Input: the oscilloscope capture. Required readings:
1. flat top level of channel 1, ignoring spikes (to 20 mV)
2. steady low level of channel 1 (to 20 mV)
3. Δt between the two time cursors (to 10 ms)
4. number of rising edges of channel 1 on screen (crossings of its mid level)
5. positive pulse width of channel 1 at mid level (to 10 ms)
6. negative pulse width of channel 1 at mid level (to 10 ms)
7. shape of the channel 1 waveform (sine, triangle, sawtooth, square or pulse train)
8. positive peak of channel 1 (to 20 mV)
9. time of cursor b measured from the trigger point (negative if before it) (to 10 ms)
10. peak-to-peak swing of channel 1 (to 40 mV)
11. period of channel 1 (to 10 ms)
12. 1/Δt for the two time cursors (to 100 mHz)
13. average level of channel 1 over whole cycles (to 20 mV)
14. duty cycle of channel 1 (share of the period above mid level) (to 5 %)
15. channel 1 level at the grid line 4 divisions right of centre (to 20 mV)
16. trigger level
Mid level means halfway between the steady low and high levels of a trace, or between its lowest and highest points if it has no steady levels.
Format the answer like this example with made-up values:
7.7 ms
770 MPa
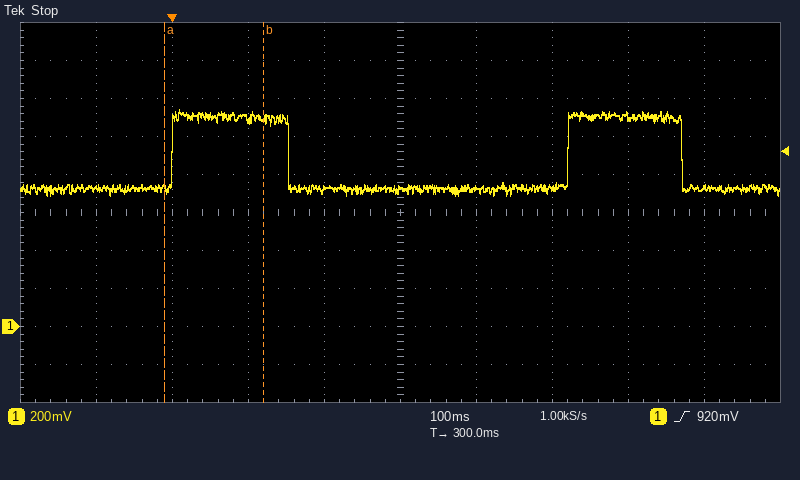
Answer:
1.10 V
720 mV
130 ms
2
150 ms
370 ms
pulse train
1.14 V
+120 ms
440 mV
520 ms
7.7 Hz
840 mV
30 %
740 mV
920 mV
